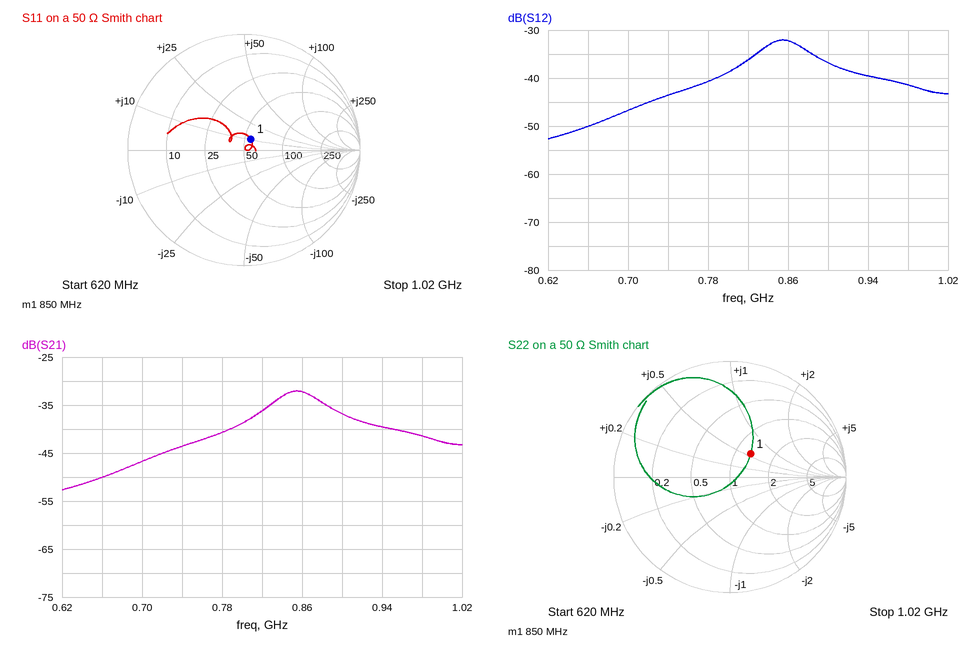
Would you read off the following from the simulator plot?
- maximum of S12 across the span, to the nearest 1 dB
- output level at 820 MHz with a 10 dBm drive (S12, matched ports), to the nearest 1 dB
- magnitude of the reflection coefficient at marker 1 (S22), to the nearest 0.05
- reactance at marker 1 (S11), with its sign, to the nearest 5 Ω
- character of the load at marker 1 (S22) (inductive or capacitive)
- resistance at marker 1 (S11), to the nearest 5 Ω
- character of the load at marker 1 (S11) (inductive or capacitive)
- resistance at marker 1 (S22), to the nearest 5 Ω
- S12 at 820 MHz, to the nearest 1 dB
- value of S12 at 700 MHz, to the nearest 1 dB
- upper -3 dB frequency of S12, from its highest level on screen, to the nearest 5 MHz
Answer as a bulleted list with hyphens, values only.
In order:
- -32 dB
- -26 dBm
- 0.25
- +10 Ω
- inductive
- 55 Ω
- inductive
- 65 Ω
- -36 dB
- -47 dB
- 885 MHz
